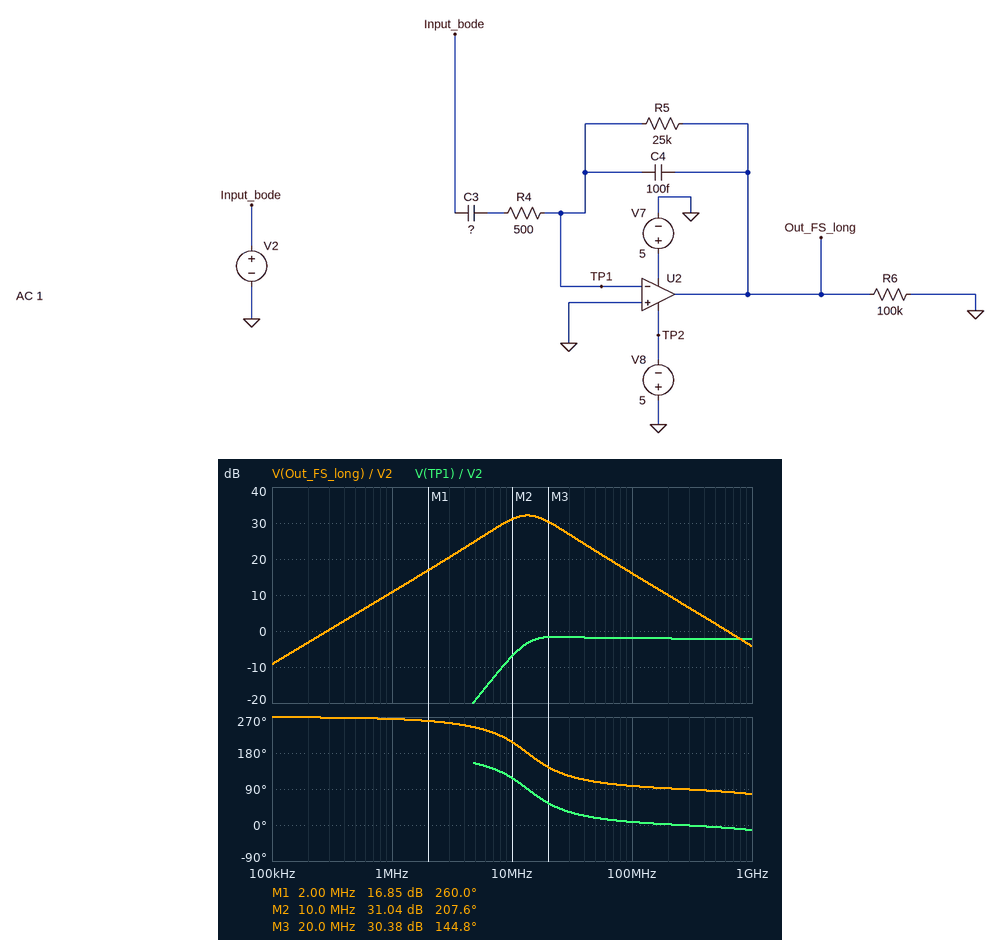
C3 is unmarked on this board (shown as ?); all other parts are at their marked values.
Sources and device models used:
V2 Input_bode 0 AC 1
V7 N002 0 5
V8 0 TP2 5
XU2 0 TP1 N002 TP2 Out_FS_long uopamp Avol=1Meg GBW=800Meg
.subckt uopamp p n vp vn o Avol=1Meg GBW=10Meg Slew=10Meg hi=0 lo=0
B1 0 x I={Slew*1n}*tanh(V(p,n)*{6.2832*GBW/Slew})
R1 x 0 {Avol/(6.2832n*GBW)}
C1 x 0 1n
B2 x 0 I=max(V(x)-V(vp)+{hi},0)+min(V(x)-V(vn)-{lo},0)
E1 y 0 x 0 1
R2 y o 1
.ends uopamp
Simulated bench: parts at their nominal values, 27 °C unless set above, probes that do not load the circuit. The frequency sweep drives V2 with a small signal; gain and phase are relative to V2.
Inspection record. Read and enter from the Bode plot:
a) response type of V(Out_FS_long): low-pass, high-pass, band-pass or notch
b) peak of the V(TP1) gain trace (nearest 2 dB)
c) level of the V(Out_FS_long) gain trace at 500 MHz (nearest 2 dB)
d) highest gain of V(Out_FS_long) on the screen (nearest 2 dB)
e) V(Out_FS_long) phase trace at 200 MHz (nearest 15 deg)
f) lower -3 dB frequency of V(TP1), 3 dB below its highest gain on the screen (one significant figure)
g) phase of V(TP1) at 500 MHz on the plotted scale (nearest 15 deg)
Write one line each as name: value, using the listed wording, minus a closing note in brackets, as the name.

response type of V(Out_FS_long): low-pass, high-pass, band-pass or notch: band-pass
peak of the V(TP1) gain trace: -2 dB
level of the V(Out_FS_long) gain trace at 500 MHz: 2 dB
highest gain of V(Out_FS_long) on the screen: 32 dB
V(Out_FS_long) phase trace at 200 MHz: 90 deg
lower -3 dB frequency of V(TP1), 3 dB below its highest gain on the screen: 10 MHz
phase of V(TP1) at 500 MHz on the plotted scale: 0 deg
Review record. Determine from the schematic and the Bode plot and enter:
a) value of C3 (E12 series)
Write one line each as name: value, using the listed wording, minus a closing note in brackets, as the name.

value of C3: 22 pF
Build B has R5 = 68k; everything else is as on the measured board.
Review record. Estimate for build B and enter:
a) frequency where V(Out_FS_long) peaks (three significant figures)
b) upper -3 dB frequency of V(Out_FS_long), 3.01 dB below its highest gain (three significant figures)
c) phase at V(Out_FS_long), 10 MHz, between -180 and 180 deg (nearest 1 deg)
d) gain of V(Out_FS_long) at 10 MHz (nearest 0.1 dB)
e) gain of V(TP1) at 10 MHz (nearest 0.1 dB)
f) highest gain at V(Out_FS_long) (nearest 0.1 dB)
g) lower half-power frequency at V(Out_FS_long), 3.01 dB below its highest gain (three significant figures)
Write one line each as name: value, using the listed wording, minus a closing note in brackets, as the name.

frequency where V(Out_FS_long) peaks: 8.22 MHz
upper -3 dB frequency of V(Out_FS_long), 3.01 dB below its highest gain: 12.9 MHz
phase at V(Out_FS_long), 10 MHz, between -180 and 180 deg: 157 deg
gain of V(Out_FS_long) at 10 MHz: 37.7 dB
gain of V(TP1) at 10 MHz: -0.4 dB
highest gain at V(Out_FS_long): 38.4 dB
lower half-power frequency at V(Out_FS_long), 3.01 dB below its highest gain: 5.25 MHz
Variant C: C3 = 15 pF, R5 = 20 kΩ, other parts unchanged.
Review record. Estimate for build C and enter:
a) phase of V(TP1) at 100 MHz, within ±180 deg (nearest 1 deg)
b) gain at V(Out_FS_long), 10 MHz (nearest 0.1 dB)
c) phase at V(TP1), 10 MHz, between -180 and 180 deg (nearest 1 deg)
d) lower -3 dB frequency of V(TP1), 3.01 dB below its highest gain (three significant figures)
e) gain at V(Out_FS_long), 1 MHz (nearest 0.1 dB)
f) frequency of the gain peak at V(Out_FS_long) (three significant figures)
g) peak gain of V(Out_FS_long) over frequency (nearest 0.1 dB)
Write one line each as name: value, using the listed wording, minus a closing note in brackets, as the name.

phase of V(TP1) at 100 MHz, within ±180 deg: 10 deg
gain at V(Out_FS_long), 10 MHz: 26.2 dB
phase at V(TP1), 10 MHz, between -180 and 180 deg: 139 deg
lower -3 dB frequency of V(TP1), 3.01 dB below its highest gain: 15.9 MHz
gain at V(Out_FS_long), 1 MHz: 5.5 dB
frequency of the gain peak at V(Out_FS_long): 18.2 MHz
peak gain of V(Out_FS_long) over frequency: 29.8 dB
